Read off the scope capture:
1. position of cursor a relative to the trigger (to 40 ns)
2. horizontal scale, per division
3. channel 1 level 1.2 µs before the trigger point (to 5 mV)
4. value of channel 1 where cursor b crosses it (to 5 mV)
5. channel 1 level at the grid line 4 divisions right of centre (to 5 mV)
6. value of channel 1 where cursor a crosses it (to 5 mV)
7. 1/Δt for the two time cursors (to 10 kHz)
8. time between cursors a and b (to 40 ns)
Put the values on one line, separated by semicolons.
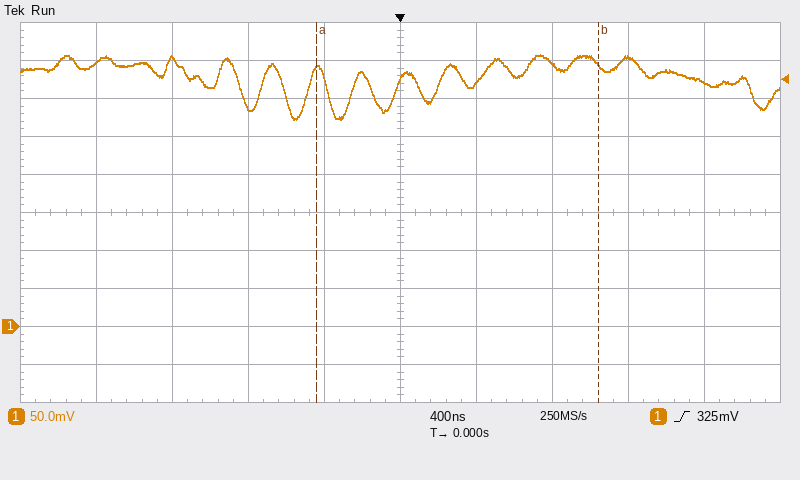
-440 ns; 400 ns; 350 mV; 345 mV; 320 mV; 340 mV; 680 kHz; 1.48 µs
